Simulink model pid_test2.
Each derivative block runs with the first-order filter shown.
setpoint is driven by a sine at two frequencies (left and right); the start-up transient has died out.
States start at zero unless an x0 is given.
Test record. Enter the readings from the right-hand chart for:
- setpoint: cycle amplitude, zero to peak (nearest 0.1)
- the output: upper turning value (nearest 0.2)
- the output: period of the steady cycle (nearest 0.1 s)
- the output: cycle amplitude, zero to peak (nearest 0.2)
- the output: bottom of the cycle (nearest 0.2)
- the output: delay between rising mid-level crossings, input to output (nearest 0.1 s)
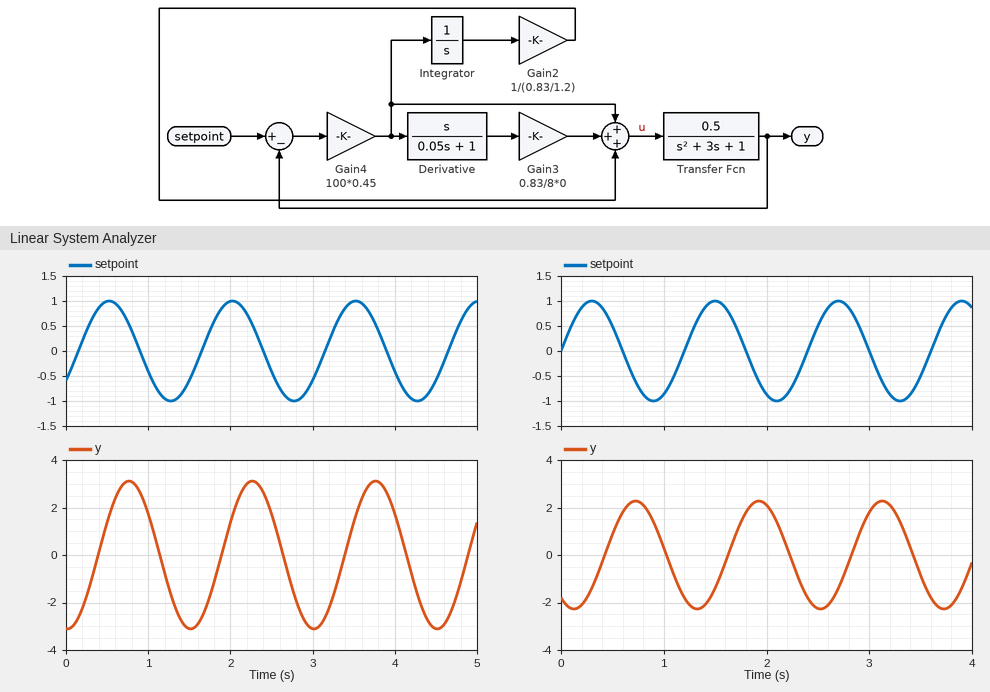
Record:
1.0
2.2
1.2 s
2.2
-2.2
0.4 s
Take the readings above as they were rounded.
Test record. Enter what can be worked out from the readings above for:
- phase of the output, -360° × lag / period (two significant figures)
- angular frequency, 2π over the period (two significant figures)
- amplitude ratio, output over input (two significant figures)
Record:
-120°
5.2 rad/s
2.2
